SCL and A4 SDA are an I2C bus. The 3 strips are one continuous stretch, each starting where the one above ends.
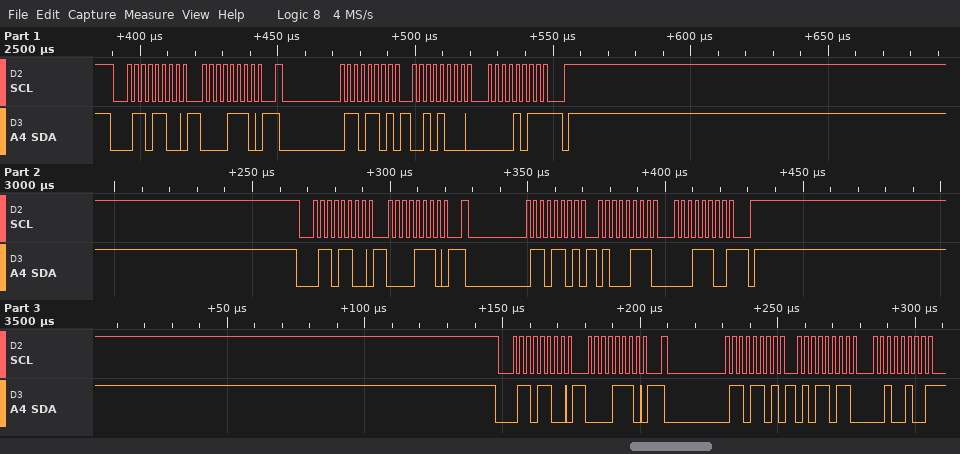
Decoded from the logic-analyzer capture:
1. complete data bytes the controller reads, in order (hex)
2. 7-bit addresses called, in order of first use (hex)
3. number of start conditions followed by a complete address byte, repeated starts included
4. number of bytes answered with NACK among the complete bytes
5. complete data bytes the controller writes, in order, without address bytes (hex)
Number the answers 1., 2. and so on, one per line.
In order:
1. 28 0B 47 1C 5B 24
2. 0x36
3. 6
4. 3
5. 0E 0E 0E
